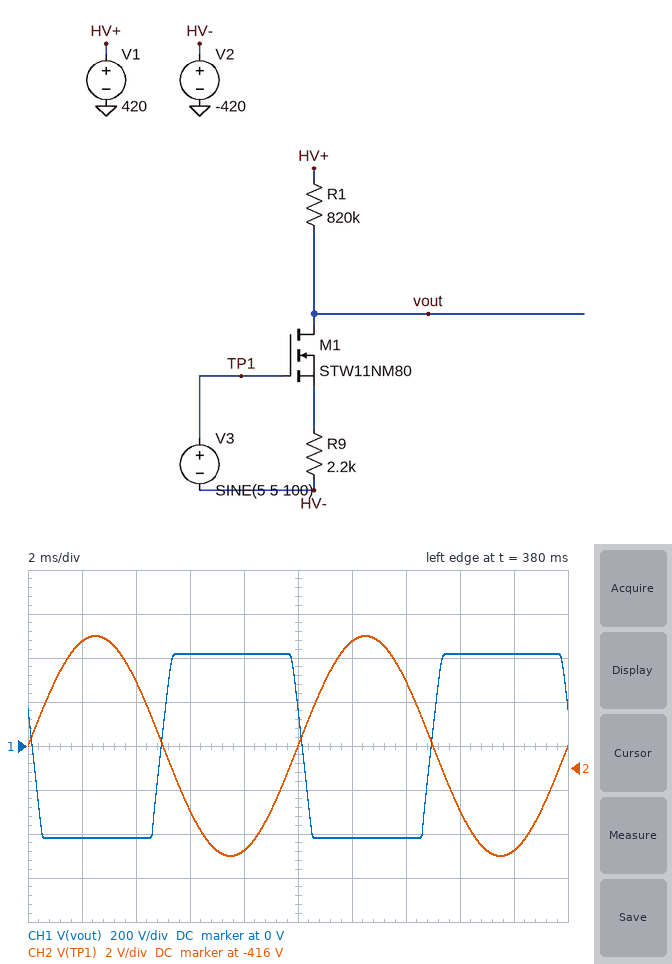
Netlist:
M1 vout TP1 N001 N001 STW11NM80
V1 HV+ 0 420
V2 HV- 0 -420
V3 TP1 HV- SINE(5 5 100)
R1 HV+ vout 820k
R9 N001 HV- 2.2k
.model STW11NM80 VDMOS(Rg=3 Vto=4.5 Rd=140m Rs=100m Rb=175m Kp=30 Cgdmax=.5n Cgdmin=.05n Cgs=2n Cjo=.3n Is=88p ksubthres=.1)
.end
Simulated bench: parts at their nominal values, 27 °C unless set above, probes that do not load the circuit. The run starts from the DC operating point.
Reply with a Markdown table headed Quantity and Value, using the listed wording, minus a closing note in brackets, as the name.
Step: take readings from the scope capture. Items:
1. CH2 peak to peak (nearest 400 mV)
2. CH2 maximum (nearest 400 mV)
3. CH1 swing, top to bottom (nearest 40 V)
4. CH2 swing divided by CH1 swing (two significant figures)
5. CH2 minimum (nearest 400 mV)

| Quantity | Value |
|---|---|
| CH2 peak to peak | 10.0 V |
| CH2 maximum | -410.0 V |
| CH1 swing, top to bottom | 840 V |
| CH2 swing divided by CH1 swing | 0.012 |
| CH2 minimum | -420.0 V |
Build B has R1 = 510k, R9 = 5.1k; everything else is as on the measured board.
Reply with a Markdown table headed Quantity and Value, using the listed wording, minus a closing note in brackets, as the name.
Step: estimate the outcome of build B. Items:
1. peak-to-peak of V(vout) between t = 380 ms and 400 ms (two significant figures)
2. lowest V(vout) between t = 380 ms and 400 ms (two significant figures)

| Quantity | Value |
|---|---|
| peak-to-peak of V(vout) between t = 380 ms and 400 ms | 570 V |
| lowest V(vout) between t = 380 ms and 400 ms | -150 V |
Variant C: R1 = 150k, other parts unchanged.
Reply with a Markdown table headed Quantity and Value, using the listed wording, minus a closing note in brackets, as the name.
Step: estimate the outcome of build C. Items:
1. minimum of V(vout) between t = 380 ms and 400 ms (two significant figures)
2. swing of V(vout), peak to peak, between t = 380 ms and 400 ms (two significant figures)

| Quantity | Value |
|---|---|
| minimum of V(vout) between t = 380 ms and 400 ms | 32 V |
| swing of V(vout), peak to peak, between t = 380 ms and 400 ms | 390 V |
